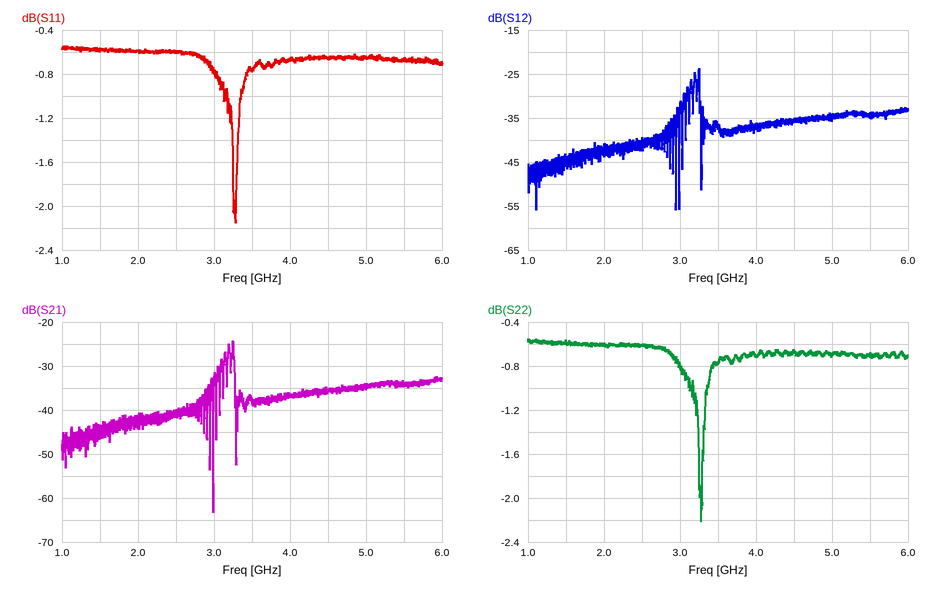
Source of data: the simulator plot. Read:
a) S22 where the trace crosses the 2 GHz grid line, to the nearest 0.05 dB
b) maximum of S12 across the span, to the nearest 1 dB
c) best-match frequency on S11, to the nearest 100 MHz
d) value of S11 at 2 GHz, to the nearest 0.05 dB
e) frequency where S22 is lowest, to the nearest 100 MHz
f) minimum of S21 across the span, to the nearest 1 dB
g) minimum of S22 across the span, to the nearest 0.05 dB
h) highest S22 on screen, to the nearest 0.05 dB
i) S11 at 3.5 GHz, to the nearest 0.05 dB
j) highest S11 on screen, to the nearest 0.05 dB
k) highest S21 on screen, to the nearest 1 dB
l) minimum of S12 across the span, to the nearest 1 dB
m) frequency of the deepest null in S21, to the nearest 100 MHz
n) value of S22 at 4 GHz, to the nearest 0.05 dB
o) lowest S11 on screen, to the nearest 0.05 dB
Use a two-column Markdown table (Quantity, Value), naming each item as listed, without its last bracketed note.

| Quantity | Value |
|---|---|
| S22 where the trace crosses the 2 GHz grid line, to the nearest 0.05 dB | -0.60 dB |
| maximum of S12 across the span, to the nearest 1 dB | -24 dB |
| best-match frequency on S11, to the nearest 100 MHz | 3.3 GHz |
| value of S11 at 2 GHz, to the nearest 0.05 dB | -0.60 dB |
| frequency where S22 is lowest, to the nearest 100 MHz | 3.3 GHz |
| minimum of S21 across the span, to the nearest 1 dB | -63 dB |
| minimum of S22 across the span, to the nearest 0.05 dB | -2.20 dB |
| highest S22 on screen, to the nearest 0.05 dB | -0.55 dB |
| S11 at 3.5 GHz, to the nearest 0.05 dB | -0.75 dB |
| highest S11 on screen, to the nearest 0.05 dB | -0.55 dB |
| highest S21 on screen, to the nearest 1 dB | -24 dB |
| minimum of S12 across the span, to the nearest 1 dB | -56 dB |
| frequency of the deepest null in S21, to the nearest 100 MHz | 3.0 GHz |
| value of S22 at 4 GHz, to the nearest 0.05 dB | -0.70 dB |
| lowest S11 on screen, to the nearest 0.05 dB | -2.15 dB |
